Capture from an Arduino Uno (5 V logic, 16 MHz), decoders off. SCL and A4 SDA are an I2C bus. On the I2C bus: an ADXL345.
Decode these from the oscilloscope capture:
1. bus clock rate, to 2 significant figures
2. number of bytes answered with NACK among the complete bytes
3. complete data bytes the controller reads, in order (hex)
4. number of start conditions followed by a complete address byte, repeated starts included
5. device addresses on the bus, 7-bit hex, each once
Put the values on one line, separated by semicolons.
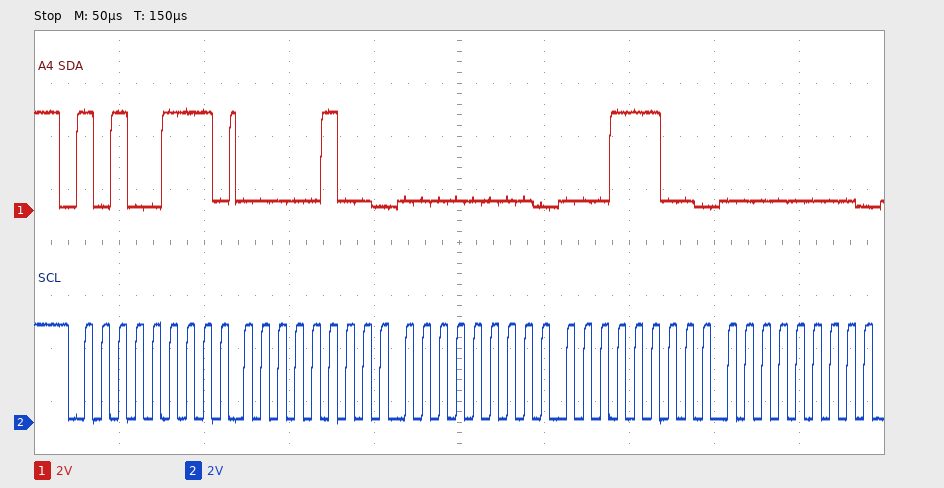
100 kHz; 0; 04 00 1C 00; 1; 0x53
